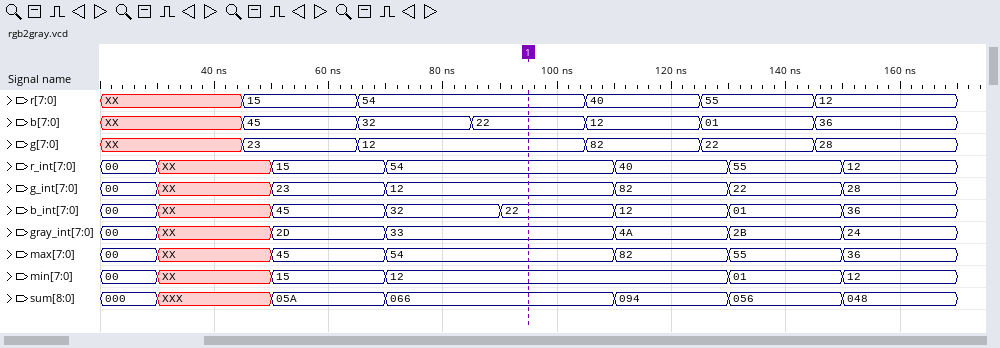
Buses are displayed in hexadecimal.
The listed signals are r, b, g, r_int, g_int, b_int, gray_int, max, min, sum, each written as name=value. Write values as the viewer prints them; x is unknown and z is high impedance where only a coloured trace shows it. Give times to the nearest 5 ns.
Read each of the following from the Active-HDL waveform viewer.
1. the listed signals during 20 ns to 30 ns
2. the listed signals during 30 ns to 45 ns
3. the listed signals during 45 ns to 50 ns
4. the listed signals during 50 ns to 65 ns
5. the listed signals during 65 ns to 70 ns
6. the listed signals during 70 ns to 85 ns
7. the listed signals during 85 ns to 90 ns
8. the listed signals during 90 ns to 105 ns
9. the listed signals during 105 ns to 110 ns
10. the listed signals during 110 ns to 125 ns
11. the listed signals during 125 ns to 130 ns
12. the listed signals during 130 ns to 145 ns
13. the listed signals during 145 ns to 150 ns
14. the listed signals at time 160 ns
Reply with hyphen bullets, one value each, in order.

- r=XX, b=XX, g=XX, r_int=00, g_int=00, b_int=00, gray_int=00, max=00, min=00, sum=000
- r=XX, b=XX, g=XX, r_int=XX, g_int=XX, b_int=XX, gray_int=XX, max=XX, min=XX, sum=XXX
- r=15, b=45, g=23, r_int=XX, g_int=XX, b_int=XX, gray_int=XX, max=XX, min=XX, sum=XXX
- r=15, b=45, g=23, r_int=15, g_int=23, b_int=45, gray_int=2D, max=45, min=15, sum=05A
- r=54, b=32, g=12, r_int=15, g_int=23, b_int=45, gray_int=2D, max=45, min=15, sum=05A
- r=54, b=32, g=12, r_int=54, g_int=12, b_int=32, gray_int=33, max=54, min=12, sum=066
- r=54, b=22, g=12, r_int=54, g_int=12, b_int=32, gray_int=33, max=54, min=12, sum=066
- r=54, b=22, g=12, r_int=54, g_int=12, b_int=22, gray_int=33, max=54, min=12, sum=066
- r=40, b=12, g=82, r_int=54, g_int=12, b_int=22, gray_int=33, max=54, min=12, sum=066
- r=40, b=12, g=82, r_int=40, g_int=82, b_int=12, gray_int=4A, max=82, min=12, sum=094
- r=55, b=01, g=22, r_int=40, g_int=82, b_int=12, gray_int=4A, max=82, min=12, sum=094
- r=55, b=01, g=22, r_int=55, g_int=22, b_int=01, gray_int=2B, max=55, min=01, sum=056
- r=12, b=36, g=28, r_int=55, g_int=22, b_int=01, gray_int=2B, max=55, min=01, sum=056
- r=12, b=36, g=28, r_int=12, g_int=28, b_int=36, gray_int=24, max=36, min=12, sum=048
